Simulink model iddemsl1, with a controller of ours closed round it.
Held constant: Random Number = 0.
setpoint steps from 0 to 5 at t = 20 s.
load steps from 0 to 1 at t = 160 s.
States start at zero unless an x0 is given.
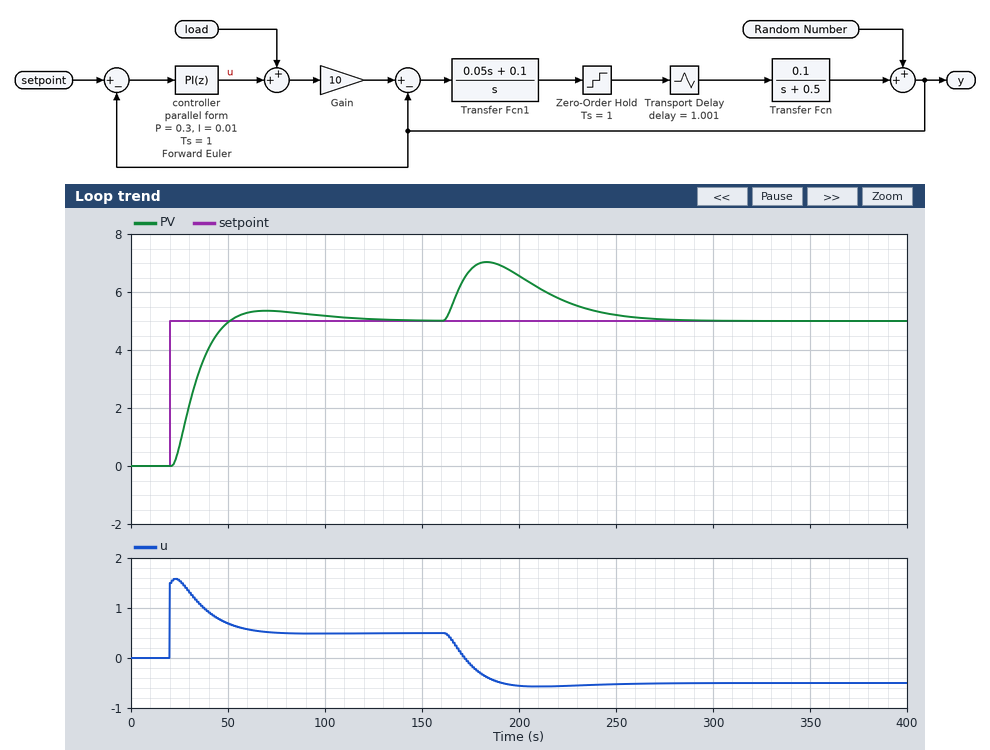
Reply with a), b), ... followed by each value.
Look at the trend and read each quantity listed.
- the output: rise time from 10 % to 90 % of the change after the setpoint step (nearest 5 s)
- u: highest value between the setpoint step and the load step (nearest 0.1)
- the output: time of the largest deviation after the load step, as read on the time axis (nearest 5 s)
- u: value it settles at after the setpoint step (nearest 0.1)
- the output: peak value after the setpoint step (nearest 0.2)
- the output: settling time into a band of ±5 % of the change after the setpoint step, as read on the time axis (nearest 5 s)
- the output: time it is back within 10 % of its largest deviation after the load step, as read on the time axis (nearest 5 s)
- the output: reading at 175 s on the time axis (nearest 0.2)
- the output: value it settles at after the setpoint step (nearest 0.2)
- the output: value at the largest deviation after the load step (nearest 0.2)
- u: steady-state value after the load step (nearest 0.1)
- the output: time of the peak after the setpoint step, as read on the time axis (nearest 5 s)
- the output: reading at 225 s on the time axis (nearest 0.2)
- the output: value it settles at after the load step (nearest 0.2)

a) 20 s
b) 1.6
c) 185 s
d) 0.5
e) 5.4
f) 90 s
g) 250 s
h) 6.8
i) 5.0
j) 7.0
k) -0.5
l) 70 s
m) 5.6
n) 5.0
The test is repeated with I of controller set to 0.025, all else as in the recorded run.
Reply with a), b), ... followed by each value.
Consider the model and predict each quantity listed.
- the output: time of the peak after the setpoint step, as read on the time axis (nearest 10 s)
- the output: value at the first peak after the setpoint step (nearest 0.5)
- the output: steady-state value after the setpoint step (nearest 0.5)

a) 50 s
b) 6.5
c) 5.0
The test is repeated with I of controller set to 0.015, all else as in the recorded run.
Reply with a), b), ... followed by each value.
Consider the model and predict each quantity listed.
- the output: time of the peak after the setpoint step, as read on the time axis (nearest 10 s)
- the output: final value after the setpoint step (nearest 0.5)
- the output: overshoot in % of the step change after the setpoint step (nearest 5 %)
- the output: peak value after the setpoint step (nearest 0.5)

a) 60 s
b) 5.0
c) 15 %
d) 6.0
